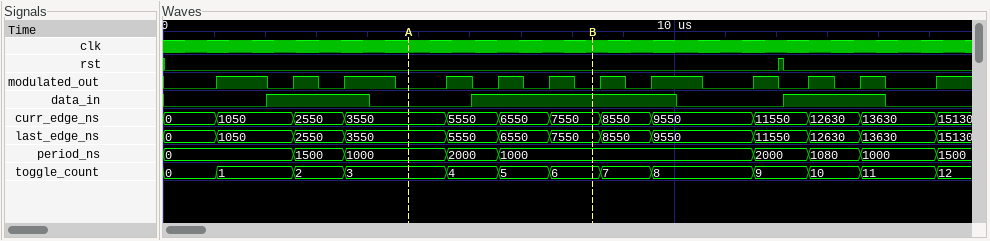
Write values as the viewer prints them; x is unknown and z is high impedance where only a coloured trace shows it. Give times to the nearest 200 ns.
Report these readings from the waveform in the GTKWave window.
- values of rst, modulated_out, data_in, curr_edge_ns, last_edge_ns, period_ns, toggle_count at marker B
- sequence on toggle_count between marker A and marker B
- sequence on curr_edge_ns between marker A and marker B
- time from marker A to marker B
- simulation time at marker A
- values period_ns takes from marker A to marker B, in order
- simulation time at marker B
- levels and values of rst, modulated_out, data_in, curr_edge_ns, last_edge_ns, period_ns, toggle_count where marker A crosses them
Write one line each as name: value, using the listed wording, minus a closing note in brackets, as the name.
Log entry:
values of rst, modulated_out, data_in, curr_edge_ns, last_edge_ns, period_ns, toggle_count at marker B: rst=0, modulated_out=0, data_in=1, curr_edge_ns=7550, last_edge_ns=7550, period_ns=1000, toggle_count=6
sequence on toggle_count between marker A and marker B: 3, 4, 5, 6
sequence on curr_edge_ns between marker A and marker B: 3550, 5550, 6550, 7550
time from marker A to marker B: 3600 ns
simulation time at marker A: 4800 ns
values period_ns takes from marker A to marker B, in order: 1000, 2000, 1000
simulation time at marker B: 8400 ns
levels and values of rst, modulated_out, data_in, curr_edge_ns, last_edge_ns, period_ns, toggle_count where marker A crosses them: rst=0, modulated_out=0, data_in=0, curr_edge_ns=3550, last_edge_ns=3550, period_ns=1000, toggle_count=3
